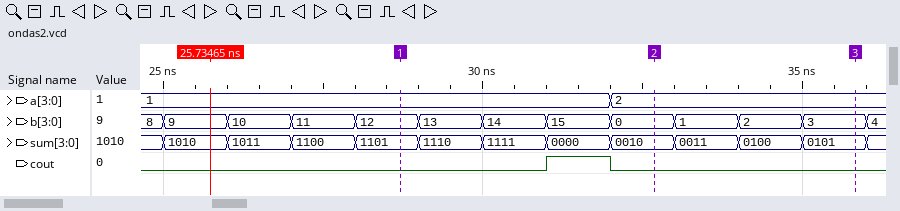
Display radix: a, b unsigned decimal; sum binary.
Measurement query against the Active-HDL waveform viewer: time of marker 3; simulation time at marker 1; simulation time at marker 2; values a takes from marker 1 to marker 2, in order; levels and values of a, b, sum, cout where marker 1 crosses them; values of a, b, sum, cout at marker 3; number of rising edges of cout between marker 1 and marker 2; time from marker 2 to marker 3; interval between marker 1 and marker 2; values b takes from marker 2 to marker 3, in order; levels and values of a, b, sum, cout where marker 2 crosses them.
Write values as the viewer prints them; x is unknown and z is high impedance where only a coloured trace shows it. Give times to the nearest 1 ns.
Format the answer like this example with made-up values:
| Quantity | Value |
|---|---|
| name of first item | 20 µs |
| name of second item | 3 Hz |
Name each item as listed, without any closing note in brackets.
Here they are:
| Quantity | Value |
|---|---|
| time of marker 3 | 36 ns |
| simulation time at marker 1 | 29 ns |
| simulation time at marker 2 | 33 ns |
| values a takes from marker 1 to marker 2, in order | 1, 2 |
| levels and values of a, b, sum, cout where marker 1 crosses them | a=1, b=12, sum=1101, cout=0 |
| values of a, b, sum, cout at marker 3 | a=2, b=3, sum=0101, cout=0 |
| number of rising edges of cout between marker 1 and marker 2 | 1 |
| time from marker 2 to marker 3 | 3 ns |
| interval between marker 1 and marker 2 | 4 ns |
| values b takes from marker 2 to marker 3, in order | 0, 1, 2, 3 |
| levels and values of a, b, sum, cout where marker 2 crosses them | a=2, b=0, sum=0010, cout=0 |
